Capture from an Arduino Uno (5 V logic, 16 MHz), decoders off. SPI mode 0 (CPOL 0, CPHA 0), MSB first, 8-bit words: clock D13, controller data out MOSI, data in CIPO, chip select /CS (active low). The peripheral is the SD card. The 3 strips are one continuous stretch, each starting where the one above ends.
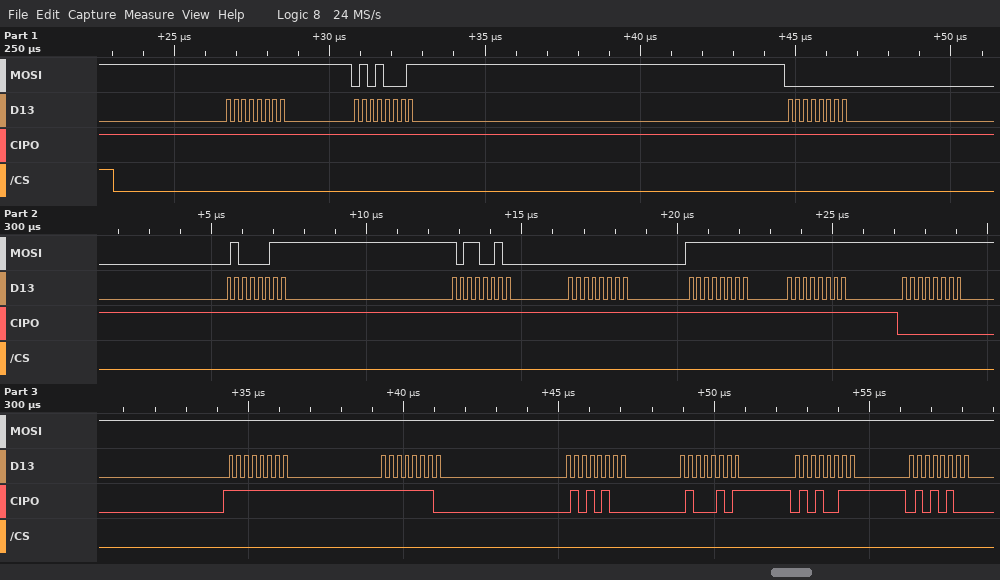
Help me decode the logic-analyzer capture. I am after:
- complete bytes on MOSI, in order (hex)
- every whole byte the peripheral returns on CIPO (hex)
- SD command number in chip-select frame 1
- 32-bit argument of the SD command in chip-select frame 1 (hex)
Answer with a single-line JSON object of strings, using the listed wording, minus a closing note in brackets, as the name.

{"complete bytes on MOSI, in order": "0xFF 0x51 0x00 0x43 0xB2 0x00 0xFF 0xFF 0xFF 0xFF 0xFF 0xFF 0xFF 0xFF 0xFF", "every whole byte the peripheral returns on CIPO": "0xFF 0xFF 0xFF 0xFF 0xFF 0xFF 0xFF 0xFF 0x00 0xFF 0xFE 0x54 0x45 0x53 0x54", "SD command number in chip-select frame 1": "CMD17", "32-bit argument of the SD command in chip-select frame 1": "0x0043B200"}
